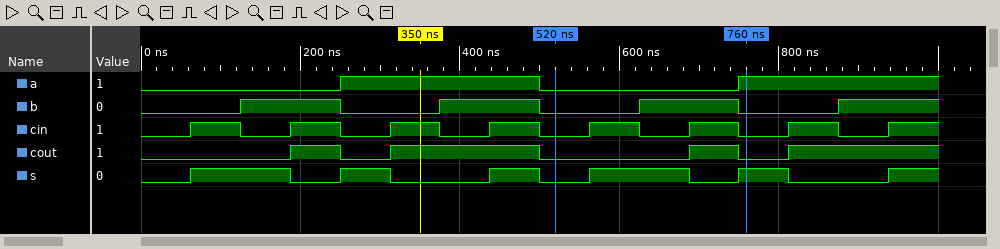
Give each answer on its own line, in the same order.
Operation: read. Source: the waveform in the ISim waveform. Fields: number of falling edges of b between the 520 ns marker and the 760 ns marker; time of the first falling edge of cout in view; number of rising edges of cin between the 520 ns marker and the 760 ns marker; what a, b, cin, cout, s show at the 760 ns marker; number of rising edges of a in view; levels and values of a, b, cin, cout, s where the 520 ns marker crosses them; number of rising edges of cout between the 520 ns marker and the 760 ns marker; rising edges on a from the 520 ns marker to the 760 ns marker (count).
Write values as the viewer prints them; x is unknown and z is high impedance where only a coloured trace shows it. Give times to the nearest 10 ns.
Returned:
1
250 ns
2
a=1, b=0, cin=0, cout=0, s=1
2
a=0, b=0, cin=0, cout=0, s=0
1
1
